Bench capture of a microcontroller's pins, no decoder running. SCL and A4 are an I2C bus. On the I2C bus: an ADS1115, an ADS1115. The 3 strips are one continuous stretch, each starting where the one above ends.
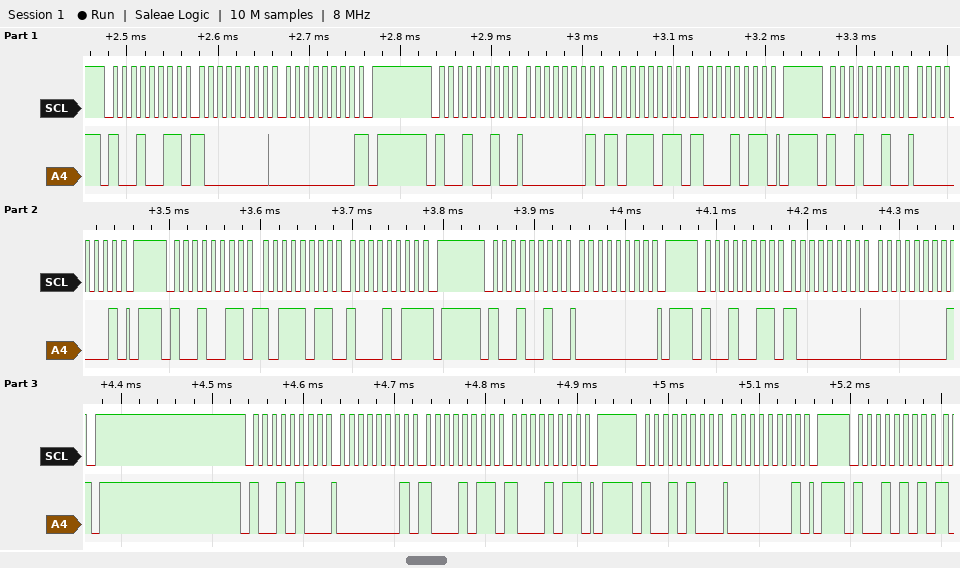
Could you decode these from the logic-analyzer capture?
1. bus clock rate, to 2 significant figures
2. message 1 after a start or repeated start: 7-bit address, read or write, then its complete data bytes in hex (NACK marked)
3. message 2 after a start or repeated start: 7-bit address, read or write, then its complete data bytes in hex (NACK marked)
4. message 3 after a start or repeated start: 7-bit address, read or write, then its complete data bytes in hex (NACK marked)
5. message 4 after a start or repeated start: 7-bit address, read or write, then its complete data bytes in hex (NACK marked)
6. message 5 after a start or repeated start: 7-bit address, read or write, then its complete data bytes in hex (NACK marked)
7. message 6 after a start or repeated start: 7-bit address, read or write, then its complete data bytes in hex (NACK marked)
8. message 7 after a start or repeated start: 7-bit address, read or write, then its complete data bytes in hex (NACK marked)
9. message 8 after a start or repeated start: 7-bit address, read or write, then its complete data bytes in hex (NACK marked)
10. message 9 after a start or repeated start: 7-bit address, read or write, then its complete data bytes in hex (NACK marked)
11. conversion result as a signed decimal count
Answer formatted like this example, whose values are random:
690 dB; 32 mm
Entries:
100 kHz; 0x49 read: 80 00 NACK; 0x49 write: 01 BB 8B; 0x49 write: 01; 0x49 read: BB 8B NACK; 0x49 write: 00; 0x49 read: 80 00 NACK; 0x4A write: 01 8B 8B; 0x4A write: 01; 0x4A read; -32768
